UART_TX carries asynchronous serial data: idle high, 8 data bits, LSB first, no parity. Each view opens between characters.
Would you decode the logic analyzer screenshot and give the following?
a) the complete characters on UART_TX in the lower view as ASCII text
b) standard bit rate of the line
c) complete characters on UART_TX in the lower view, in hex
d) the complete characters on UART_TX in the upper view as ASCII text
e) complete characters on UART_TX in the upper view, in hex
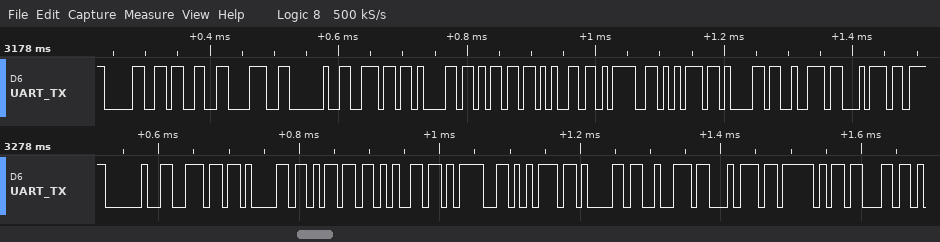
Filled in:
" name=uart_c"
115200 baud
20, 6E, 61, 6D, 65, 3D, 75, 61, 72, 74, 5F, 63
"038 name=uart"
30, 33, 38, 20, 6E, 61, 6D, 65, 3D, 75, 61, 72, 74
